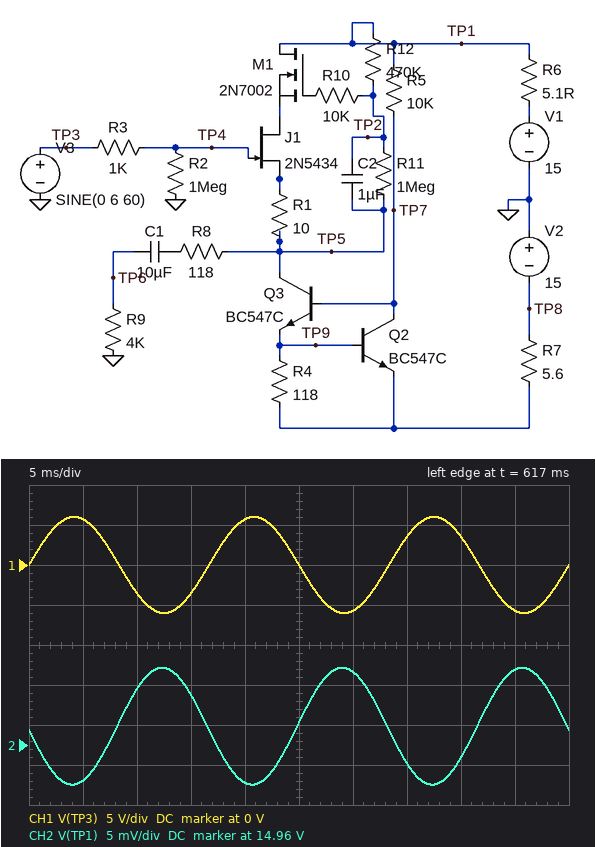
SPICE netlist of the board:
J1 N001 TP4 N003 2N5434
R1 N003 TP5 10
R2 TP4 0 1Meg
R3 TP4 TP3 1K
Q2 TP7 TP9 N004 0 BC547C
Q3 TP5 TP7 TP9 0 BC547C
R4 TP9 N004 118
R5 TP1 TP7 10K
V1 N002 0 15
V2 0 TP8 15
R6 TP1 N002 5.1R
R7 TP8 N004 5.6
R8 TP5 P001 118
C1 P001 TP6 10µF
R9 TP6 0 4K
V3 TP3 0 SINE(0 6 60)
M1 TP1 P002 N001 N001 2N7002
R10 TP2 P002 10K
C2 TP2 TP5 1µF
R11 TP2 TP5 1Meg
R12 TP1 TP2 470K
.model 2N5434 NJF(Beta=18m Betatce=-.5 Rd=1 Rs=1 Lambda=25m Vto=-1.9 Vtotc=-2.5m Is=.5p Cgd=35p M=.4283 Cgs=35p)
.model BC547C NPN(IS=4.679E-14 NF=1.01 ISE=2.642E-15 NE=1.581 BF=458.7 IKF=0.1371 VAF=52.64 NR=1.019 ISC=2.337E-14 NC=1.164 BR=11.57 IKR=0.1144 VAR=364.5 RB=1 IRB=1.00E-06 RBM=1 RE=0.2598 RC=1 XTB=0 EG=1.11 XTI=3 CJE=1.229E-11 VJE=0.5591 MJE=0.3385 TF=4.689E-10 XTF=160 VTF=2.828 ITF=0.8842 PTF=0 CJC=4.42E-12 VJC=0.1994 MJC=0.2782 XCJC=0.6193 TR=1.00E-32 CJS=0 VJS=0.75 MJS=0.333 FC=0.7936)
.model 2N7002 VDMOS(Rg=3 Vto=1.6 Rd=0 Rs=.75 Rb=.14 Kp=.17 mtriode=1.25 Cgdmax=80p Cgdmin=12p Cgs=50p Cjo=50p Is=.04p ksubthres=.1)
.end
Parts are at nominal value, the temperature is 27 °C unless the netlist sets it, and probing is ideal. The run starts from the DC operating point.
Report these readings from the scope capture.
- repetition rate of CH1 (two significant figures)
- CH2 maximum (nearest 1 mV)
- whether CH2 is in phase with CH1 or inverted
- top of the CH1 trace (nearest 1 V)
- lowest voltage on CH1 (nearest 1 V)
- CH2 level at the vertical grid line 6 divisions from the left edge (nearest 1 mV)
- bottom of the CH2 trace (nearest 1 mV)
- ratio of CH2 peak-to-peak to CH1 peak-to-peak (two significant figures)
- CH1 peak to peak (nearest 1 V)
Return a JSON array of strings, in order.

["60 Hz", "14.965 V", "inverted", "6 V", "-6 V", "14.964 V", "14.950 V", "0.0012", "12 V"]
